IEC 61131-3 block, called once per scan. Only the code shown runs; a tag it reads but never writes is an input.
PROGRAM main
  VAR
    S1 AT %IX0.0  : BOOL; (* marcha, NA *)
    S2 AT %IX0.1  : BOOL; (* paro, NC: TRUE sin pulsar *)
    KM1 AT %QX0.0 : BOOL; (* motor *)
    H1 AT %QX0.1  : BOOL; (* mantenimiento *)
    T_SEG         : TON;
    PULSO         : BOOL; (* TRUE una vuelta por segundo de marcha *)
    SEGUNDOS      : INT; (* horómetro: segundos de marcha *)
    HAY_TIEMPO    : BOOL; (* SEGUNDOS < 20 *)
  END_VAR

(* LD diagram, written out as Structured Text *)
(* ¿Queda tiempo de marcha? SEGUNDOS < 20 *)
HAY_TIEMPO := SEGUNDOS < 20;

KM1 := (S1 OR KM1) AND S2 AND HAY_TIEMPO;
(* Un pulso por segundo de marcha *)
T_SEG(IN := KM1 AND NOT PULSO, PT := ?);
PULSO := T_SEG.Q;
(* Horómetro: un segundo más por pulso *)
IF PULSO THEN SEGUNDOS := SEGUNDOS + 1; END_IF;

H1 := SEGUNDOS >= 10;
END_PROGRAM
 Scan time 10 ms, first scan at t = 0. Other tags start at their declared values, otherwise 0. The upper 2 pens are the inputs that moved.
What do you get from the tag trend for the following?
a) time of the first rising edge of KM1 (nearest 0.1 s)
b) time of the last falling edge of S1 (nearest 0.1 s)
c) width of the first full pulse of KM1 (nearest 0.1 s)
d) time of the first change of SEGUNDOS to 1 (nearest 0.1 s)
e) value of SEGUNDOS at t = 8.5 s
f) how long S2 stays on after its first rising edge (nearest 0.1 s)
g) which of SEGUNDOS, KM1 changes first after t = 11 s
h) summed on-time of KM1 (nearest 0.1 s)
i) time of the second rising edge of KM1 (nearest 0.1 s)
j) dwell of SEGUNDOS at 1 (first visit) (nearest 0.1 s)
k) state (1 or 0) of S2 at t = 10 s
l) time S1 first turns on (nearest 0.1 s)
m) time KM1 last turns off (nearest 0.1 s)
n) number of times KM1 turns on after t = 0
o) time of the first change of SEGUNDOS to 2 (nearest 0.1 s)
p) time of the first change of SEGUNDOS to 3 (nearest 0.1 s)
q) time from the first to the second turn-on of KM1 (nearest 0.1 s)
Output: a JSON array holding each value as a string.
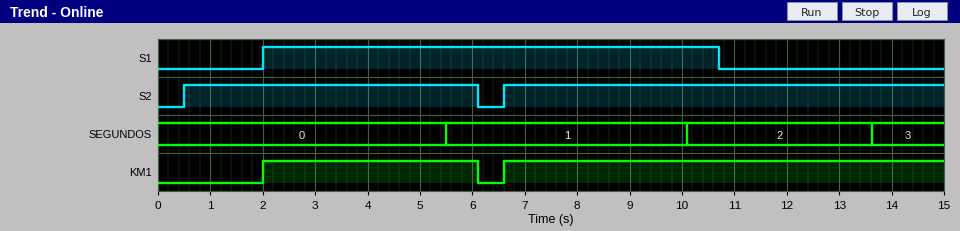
["2.0 s", "10.7 s", "4.1 s", "5.5 s", "1", "5.6 s", "SEGUNDOS", "12.5 s", "6.6 s", "4.6 s", "1", "2.0 s", "6.1 s", "2", "10.1 s", "13.6 s", "4.6 s"]
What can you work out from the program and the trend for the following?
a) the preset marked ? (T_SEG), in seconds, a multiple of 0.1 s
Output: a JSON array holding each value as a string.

["3.5 s"]
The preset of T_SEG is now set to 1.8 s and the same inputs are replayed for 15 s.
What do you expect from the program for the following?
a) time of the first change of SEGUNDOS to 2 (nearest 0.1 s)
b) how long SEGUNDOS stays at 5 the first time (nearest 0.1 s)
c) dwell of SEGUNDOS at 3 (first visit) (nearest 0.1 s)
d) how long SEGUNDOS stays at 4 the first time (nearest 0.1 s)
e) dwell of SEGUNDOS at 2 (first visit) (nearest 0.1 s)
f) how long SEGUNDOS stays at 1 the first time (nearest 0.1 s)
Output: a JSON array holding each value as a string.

["5.6 s", "1.8 s", "1.8 s", "1.8 s", "2.8 s", "1.8 s"]
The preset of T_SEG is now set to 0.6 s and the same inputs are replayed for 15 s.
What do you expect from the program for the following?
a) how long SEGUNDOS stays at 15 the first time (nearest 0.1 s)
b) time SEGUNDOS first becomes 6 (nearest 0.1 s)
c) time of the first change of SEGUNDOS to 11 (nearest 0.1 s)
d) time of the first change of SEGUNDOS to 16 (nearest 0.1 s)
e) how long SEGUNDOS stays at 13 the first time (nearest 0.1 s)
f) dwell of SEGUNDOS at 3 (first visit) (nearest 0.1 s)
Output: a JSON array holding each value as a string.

["0.6 s", "5.7 s", "9.7 s", "12.8 s", "0.6 s", "0.6 s"]
